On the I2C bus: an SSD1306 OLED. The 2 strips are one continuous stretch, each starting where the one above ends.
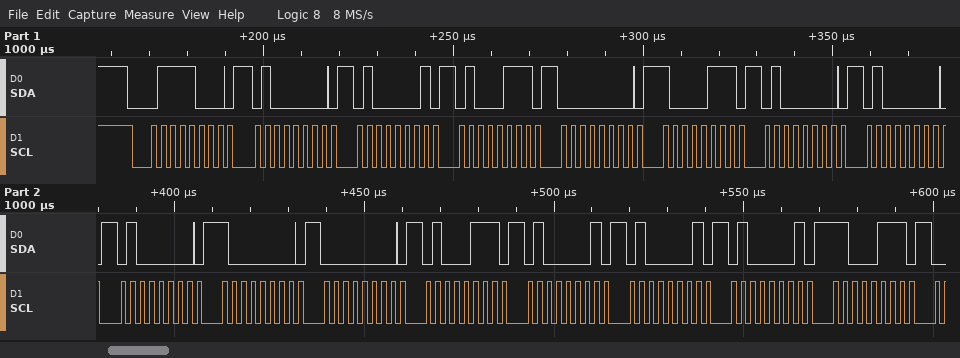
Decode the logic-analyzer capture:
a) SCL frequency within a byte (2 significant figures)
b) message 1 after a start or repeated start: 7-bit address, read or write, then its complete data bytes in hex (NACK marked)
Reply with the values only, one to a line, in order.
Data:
400 kHz
0x3C write: 40 41 47 00 87 40 40 40 80 00 47 41 41 41 C7
